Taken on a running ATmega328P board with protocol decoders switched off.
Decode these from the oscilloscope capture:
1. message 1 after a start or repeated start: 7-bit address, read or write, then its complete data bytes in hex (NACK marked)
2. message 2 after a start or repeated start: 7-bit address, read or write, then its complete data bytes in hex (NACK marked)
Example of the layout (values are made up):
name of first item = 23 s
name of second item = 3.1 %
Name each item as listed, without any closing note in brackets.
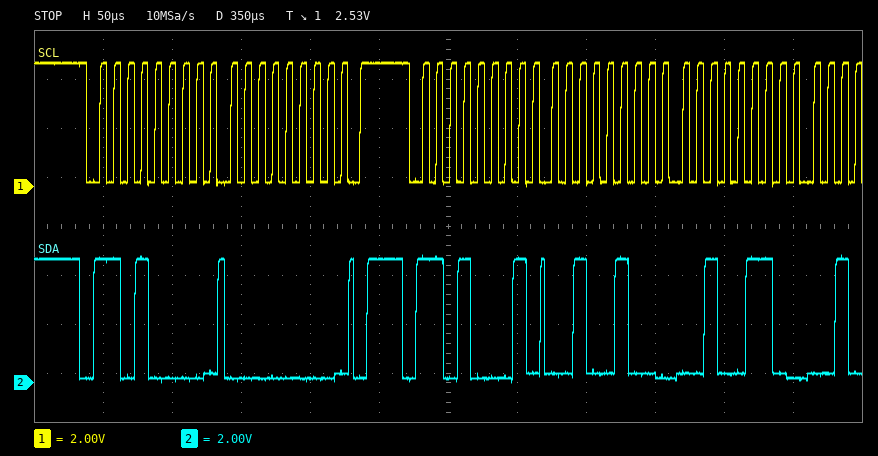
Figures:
message 1 after a start or repeated start: 7-bit address, read or write, then its complete data bytes in hex = 0x68 write: 00
message 2 after a start or repeated start: 7-bit address, read or write, then its complete data bytes in hex = 0x68 read: 24 26
